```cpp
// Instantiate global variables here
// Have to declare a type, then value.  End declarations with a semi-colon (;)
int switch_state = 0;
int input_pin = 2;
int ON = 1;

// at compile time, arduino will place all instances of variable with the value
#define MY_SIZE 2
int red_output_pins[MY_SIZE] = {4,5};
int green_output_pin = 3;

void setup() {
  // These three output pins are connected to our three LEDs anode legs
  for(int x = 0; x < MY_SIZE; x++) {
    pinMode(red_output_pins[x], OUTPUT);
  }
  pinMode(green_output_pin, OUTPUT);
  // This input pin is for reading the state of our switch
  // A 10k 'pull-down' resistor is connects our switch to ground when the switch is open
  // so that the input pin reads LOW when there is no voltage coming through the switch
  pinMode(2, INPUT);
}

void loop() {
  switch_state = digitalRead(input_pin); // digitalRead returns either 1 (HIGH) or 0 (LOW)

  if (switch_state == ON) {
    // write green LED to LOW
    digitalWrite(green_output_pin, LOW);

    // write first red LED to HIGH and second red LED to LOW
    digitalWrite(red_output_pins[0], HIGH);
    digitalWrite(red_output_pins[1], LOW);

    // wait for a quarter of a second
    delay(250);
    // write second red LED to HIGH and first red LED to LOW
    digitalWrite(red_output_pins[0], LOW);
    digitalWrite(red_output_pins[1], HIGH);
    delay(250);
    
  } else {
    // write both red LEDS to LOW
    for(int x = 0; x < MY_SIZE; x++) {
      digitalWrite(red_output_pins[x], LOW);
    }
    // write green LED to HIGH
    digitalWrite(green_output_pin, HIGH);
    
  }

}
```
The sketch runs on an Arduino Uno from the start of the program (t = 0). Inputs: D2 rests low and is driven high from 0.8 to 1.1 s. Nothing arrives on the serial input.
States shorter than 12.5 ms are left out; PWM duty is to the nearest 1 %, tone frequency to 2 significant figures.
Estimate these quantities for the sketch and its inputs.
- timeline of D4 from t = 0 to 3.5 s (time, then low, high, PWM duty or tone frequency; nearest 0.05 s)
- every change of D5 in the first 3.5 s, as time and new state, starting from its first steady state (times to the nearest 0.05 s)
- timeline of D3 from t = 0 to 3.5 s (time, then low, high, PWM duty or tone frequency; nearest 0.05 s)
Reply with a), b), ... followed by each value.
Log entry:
a) 0 s low; 0.8 s high; 1.05 s low
b) 0 s low; 1.05 s high; 1.3 s low
c) 0 s high; 0.8 s low; 1.3 s high
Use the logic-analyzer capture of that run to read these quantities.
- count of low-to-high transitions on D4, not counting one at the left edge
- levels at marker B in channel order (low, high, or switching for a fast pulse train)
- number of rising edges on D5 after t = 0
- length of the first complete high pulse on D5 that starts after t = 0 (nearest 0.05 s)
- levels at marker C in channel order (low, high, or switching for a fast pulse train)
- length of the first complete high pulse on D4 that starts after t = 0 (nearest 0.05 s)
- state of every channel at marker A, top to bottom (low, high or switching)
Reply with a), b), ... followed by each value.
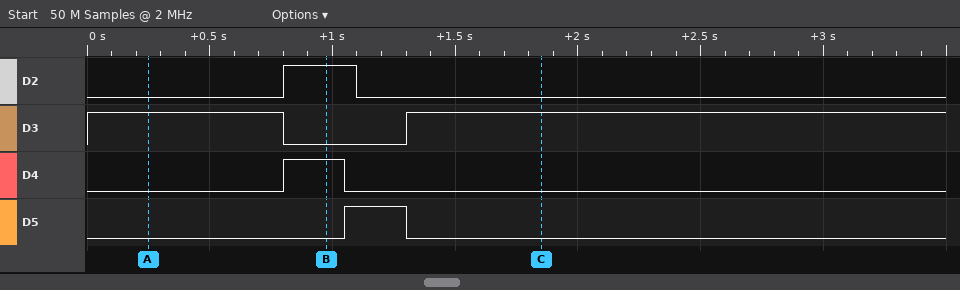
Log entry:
a) 1
b) D2 high, D3 low, D4 high, D5 low
c) 1
d) 0.25 s
e) D2 low, D3 high, D4 low, D5 low
f) 0.25 s
g) D2 low, D3 high, D4 low, D5 low
